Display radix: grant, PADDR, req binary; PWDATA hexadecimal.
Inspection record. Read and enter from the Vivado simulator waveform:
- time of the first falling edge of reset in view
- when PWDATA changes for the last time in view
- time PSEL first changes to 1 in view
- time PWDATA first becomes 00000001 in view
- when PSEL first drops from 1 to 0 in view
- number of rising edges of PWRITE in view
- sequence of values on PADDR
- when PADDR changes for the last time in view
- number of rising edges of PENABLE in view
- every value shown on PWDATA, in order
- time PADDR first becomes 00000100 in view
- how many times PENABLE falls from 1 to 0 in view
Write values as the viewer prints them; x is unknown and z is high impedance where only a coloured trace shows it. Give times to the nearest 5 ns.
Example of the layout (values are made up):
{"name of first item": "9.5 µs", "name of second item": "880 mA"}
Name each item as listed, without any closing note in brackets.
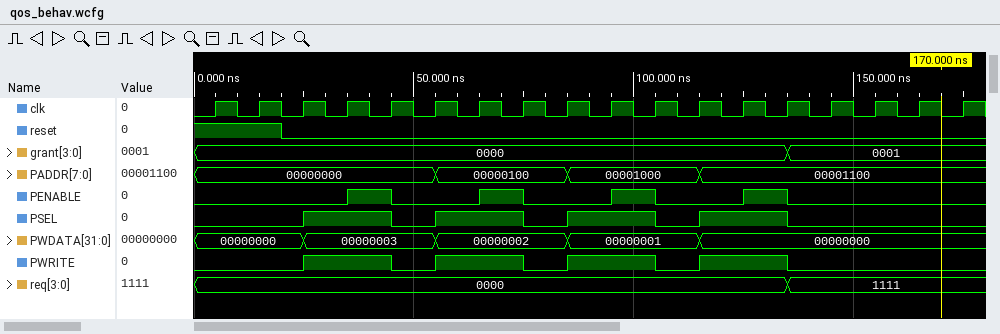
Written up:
{"time of the first falling edge of reset in view": "20 ns", "when PWDATA changes for the last time in view": "115 ns", "time PSEL first changes to 1 in view": "25 ns", "time PWDATA first becomes 00000001 in view": "85 ns", "when PSEL first drops from 1 to 0 in view": "45 ns", "number of rising edges of PWRITE in view": "4", "sequence of values on PADDR": "00000000, 00000100, 00001000, 00001100", "when PADDR changes for the last time in view": "115 ns", "number of rising edges of PENABLE in view": "4", "every value shown on PWDATA, in order": "00000000, 00000003, 00000002, 00000001, 00000000", "time PADDR first becomes 00000100 in view": "55 ns", "how many times PENABLE falls from 1 to 0 in view": "4"}
